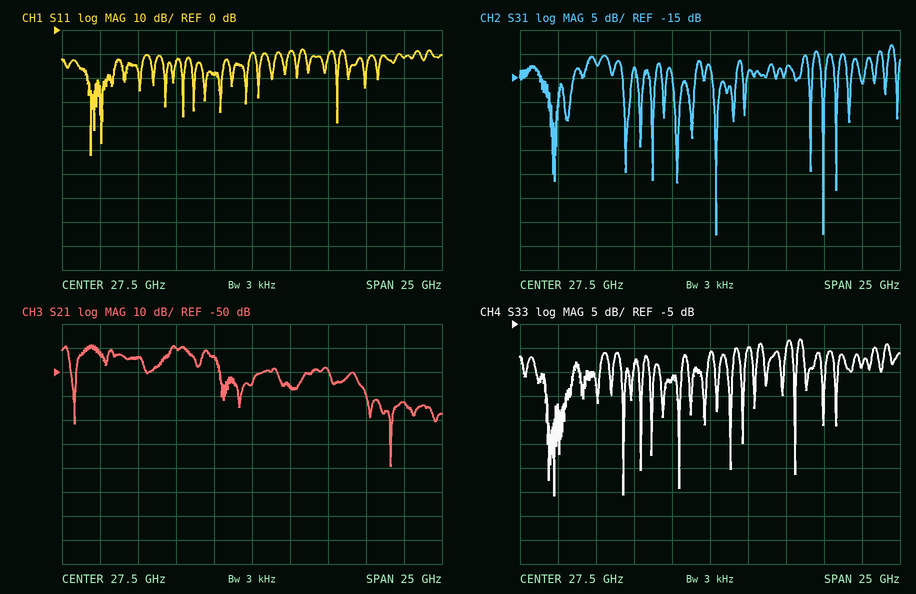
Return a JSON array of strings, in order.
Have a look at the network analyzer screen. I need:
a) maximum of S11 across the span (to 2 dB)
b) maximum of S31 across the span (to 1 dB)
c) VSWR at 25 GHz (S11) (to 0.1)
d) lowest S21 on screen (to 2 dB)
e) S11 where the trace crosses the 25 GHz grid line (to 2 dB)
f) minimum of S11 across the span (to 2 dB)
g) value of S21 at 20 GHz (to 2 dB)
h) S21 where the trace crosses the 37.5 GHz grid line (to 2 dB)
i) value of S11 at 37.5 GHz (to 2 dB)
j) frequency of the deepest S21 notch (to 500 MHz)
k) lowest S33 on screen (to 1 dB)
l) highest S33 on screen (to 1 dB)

["-8 dB", "-8 dB", "1.3", "-90 dB", "-18 dB", "-52 dB", "-44 dB", "-62 dB", "-12 dB", "36.5 GHz", "-41 dB", "-8 dB"]
